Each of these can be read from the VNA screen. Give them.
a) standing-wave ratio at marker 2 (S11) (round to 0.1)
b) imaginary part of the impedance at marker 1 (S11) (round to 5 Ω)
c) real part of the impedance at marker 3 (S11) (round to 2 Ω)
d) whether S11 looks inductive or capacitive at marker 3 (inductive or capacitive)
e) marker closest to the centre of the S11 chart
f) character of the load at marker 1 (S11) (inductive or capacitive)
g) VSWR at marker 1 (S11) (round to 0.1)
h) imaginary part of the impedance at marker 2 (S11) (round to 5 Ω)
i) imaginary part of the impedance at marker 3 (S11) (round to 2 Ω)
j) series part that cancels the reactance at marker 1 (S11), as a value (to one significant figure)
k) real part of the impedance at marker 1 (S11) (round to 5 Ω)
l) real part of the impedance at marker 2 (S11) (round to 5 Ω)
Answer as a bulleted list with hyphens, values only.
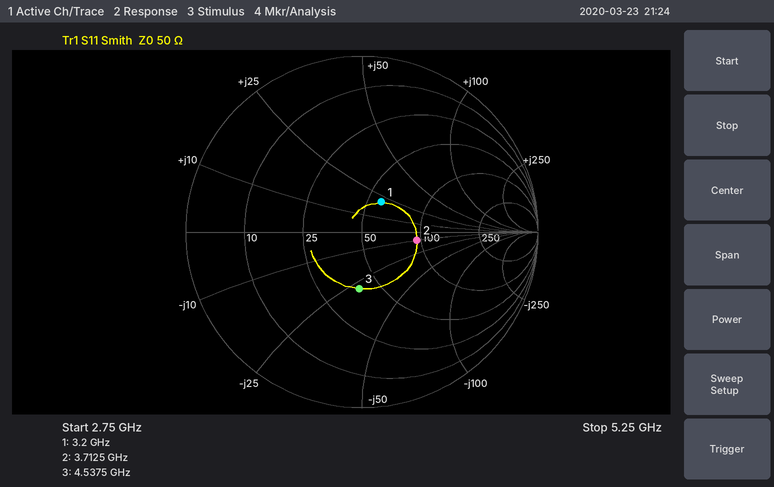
- 1.9
- +20 Ω
- 40 Ω
- capacitive
- marker 1
- inductive
- 1.5
- -10 Ω
- -28 Ω
- 2 pF
- 60 Ω
- 95 Ω
